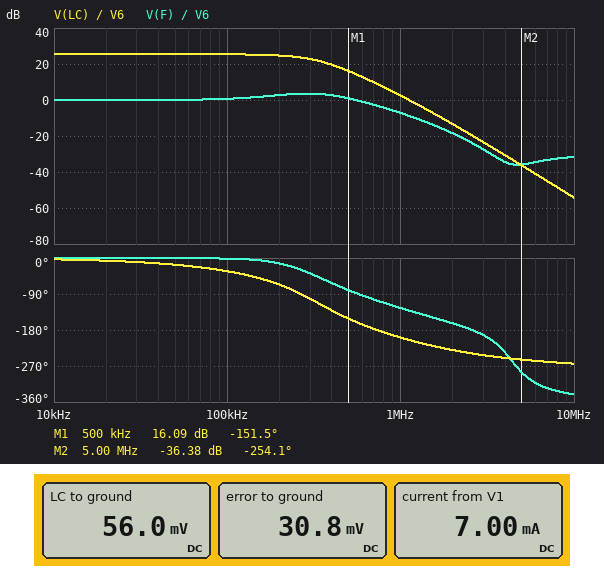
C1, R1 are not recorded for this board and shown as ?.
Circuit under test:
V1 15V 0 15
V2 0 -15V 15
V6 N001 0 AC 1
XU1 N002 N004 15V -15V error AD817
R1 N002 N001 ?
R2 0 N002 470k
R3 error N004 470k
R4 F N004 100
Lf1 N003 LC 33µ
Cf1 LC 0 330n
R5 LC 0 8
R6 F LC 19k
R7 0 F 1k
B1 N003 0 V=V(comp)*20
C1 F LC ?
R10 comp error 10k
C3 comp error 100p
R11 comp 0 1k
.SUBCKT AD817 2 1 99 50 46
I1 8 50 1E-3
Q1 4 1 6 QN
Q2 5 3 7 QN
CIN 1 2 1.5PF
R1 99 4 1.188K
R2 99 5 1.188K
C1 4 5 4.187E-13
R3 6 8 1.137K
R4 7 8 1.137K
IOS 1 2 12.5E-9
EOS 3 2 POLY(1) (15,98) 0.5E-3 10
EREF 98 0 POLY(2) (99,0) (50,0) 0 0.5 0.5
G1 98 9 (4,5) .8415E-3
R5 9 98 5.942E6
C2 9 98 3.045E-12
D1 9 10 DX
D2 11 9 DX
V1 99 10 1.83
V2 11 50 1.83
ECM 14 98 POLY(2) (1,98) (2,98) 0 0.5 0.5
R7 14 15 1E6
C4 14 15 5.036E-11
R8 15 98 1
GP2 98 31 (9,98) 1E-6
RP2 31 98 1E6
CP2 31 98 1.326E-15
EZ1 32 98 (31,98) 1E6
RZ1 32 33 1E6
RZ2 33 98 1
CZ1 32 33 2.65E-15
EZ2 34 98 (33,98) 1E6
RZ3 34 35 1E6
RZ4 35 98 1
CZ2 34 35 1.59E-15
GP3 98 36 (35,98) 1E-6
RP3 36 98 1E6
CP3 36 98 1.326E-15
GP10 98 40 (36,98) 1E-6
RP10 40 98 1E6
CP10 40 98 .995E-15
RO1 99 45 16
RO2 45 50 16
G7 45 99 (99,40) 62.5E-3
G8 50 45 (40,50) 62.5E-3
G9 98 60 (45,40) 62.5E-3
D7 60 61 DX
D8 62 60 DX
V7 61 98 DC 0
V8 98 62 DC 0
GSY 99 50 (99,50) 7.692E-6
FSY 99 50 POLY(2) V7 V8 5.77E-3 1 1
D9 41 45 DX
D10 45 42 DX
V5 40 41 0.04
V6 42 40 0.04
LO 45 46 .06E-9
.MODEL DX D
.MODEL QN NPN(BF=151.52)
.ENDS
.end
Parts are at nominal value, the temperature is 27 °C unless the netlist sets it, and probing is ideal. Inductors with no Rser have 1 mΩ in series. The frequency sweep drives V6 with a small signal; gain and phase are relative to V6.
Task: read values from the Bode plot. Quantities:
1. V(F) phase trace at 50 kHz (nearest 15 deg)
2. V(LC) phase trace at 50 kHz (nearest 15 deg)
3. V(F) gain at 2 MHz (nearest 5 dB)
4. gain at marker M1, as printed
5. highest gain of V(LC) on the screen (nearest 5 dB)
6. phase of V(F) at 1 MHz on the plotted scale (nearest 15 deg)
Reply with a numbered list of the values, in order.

1. 0 deg
2. -15 deg
3. -20 dB
4. 16.09 dB
5. 25 dB
6. -120 deg
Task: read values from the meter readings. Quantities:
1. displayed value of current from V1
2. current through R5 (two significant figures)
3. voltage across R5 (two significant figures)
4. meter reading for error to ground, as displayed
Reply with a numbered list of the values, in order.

1. 7.00 mA
2. 7.0 mA
3. 56 mV
4. 30.8 mV
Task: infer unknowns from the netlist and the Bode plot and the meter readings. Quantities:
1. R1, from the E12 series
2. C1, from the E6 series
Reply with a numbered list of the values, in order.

1. 330 Ω
2. 47 pF
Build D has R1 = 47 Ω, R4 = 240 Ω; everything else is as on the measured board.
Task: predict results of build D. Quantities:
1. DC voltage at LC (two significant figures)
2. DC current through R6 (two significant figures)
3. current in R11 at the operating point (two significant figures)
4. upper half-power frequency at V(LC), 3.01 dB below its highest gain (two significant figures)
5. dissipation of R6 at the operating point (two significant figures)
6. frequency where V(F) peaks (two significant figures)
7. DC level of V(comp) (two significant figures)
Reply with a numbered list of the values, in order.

1. 83 mV
2. 4.3 µA
3. 4.1 µA
4. 290 kHz
5. 350 nW
6. 280 kHz
7. 4.1 mV
